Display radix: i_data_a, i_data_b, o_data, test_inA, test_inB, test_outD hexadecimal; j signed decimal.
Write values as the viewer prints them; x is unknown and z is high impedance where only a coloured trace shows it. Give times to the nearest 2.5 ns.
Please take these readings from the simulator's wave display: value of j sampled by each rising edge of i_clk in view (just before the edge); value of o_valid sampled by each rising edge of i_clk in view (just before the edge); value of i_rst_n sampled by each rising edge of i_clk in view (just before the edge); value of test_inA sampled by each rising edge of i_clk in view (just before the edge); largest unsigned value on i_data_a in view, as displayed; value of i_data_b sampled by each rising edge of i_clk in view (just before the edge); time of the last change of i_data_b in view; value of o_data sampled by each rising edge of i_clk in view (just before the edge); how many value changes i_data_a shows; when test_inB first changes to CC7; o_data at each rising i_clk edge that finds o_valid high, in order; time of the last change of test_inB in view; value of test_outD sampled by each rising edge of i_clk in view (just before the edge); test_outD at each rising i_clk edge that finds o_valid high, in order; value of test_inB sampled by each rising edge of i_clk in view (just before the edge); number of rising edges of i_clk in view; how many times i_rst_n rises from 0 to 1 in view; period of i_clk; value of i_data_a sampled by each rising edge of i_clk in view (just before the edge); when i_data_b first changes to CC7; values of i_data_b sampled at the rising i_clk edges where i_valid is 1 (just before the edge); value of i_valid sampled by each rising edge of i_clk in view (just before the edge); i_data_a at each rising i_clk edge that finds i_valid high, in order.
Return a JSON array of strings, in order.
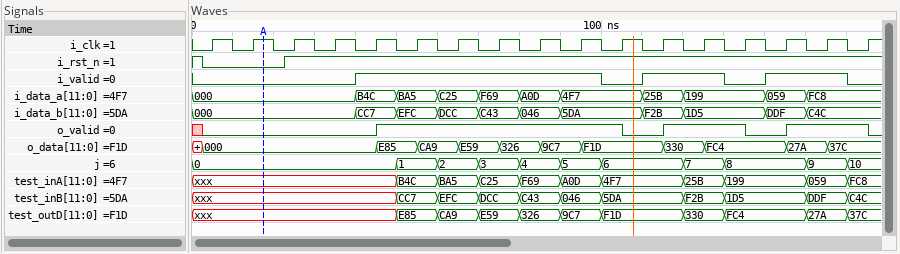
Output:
["0, 0, 0, 0, 0, 1, 2, 3, 4, 5, 6, 6, 7, 8, 8, 9, 10", "0 0 0 0 0 1 1 1 1 1 1 0 1 1 0 1 1", "0 0 1 1 1 1 1 1 1 1 1 1 1 1 1 1 1", "xxx, xxx, xxx, xxx, xxx, B4C, BA5, C25, F69, A0D, 4F7, 4F7, 25B, 199, 199, 059, FC8", "FC8", "000, 000, 000, 000, CC7, EFC, DCC, C43, 046, 5DA, 5DA, F2B, 1D5, 1D5, DDF, C4C, C4C", "150 ns", "000, 000, 000, 000, 000, E85, CA9, E59, 326, 9C7, F1D, F1D, 330, FC4, FC4, 27A, 37C", "10", "50 ns", "E85, CA9, E59, 326, 9C7, F1D, 330, FC4, 27A, 37C", "160 ns", "xxx, xxx, xxx, xxx, xxx, E85, CA9, E59, 326, 9C7, F1D, F1D, 330, FC4, FC4, 27A, 37C", "E85, CA9, E59, 326, 9C7, F1D, 330, FC4, 27A, 37C", "xxx, xxx, xxx, xxx, xxx, CC7, EFC, DCC, C43, 046, 5DA, 5DA, F2B, 1D5, 1D5, DDF, C4C", "17", "1", "10 ns", "000, 000, 000, 000, B4C, BA5, C25, F69, A0D, 4F7, 4F7, 25B, 199, 199, 059, FC8, FC8", "40 ns", "CC7, EFC, DCC, C43, 046, 5DA, F2B, 1D5, DDF, C4C", "0 0 0 0 1 1 1 1 1 1 0 1 1 0 1 1 0", "B4C, BA5, C25, F69, A0D, 4F7, 25B, 199, 059, FC8"]
